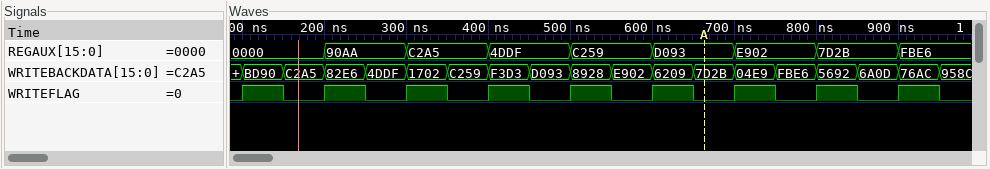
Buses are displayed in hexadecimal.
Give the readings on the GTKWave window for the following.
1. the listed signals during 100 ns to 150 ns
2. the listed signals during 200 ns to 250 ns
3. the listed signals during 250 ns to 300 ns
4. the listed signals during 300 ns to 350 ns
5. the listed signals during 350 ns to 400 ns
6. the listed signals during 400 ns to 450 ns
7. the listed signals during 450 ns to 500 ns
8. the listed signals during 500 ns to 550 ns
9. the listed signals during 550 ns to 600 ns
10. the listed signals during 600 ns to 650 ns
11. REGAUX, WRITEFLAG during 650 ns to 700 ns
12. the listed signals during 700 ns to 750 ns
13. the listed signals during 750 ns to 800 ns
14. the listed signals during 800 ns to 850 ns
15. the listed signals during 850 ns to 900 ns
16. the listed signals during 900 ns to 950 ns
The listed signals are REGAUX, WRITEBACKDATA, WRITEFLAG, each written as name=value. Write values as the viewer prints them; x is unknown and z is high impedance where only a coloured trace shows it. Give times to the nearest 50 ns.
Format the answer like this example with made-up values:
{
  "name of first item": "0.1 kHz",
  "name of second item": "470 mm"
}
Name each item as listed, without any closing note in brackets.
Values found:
{
  "the listed signals during 100 ns to 150 ns": "REGAUX=0000, WRITEBACKDATA=BD90, WRITEFLAG=1",
  "the listed signals during 200 ns to 250 ns": "REGAUX=90AA, WRITEBACKDATA=82E6, WRITEFLAG=1",
  "the listed signals during 250 ns to 300 ns": "REGAUX=90AA, WRITEBACKDATA=4DDF, WRITEFLAG=0",
  "the listed signals during 300 ns to 350 ns": "REGAUX=C2A5, WRITEBACKDATA=1702, WRITEFLAG=1",
  "the listed signals during 350 ns to 400 ns": "REGAUX=C2A5, WRITEBACKDATA=C259, WRITEFLAG=0",
  "the listed signals during 400 ns to 450 ns": "REGAUX=4DDF, WRITEBACKDATA=F3D3, WRITEFLAG=1",
  "the listed signals during 450 ns to 500 ns": "REGAUX=4DDF, WRITEBACKDATA=D093, WRITEFLAG=0",
  "the listed signals during 500 ns to 550 ns": "REGAUX=C259, WRITEBACKDATA=8928, WRITEFLAG=1",
  "the listed signals during 550 ns to 600 ns": "REGAUX=C259, WRITEBACKDATA=E902, WRITEFLAG=0",
  "the listed signals during 600 ns to 650 ns": "REGAUX=D093, WRITEBACKDATA=6209, WRITEFLAG=1",
  "REGAUX, WRITEFLAG during 650 ns to 700 ns": "REGAUX=D093, WRITEFLAG=0",
  "the listed signals during 700 ns to 750 ns": "REGAUX=E902, WRITEBACKDATA=04E9, WRITEFLAG=1",
  "the listed signals during 750 ns to 800 ns": "REGAUX=E902, WRITEBACKDATA=FBE6, WRITEFLAG=0",
  "the listed signals during 800 ns to 850 ns": "REGAUX=7D2B, WRITEBACKDATA=5692, WRITEFLAG=1",
  "the listed signals during 850 ns to 900 ns": "REGAUX=7D2B, WRITEBACKDATA=6A0D, WRITEFLAG=0",
  "the listed signals during 900 ns to 950 ns": "REGAUX=FBE6, WRITEBACKDATA=76AC, WRITEFLAG=1"
}
